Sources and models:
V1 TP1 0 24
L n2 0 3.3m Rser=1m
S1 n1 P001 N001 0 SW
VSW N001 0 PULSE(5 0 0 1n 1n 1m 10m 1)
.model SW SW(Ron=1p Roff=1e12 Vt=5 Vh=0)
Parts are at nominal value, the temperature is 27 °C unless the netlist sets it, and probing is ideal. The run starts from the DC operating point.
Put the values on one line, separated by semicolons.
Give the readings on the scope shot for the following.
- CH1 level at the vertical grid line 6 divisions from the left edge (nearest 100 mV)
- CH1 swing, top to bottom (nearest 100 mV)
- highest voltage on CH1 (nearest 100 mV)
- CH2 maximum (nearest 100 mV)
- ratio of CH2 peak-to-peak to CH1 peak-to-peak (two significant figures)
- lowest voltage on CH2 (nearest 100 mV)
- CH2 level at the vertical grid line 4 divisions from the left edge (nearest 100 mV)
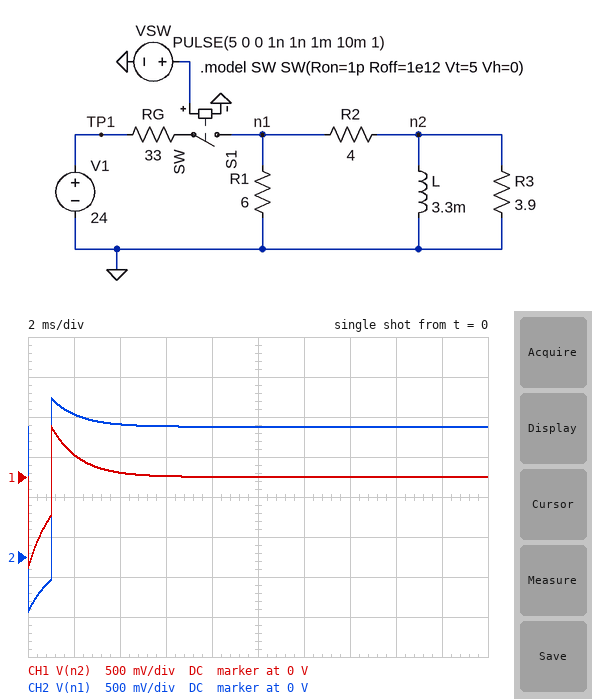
0 V; 1.8 V; 600 mV; 2.0 V; 1.5; -700 mV; 1.6 V
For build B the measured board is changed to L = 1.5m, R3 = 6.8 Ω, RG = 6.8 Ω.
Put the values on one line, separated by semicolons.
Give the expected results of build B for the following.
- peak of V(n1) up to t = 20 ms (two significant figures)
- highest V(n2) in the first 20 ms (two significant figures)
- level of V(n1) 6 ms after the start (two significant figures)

8.5 V; 5.1 V; 6.3 V
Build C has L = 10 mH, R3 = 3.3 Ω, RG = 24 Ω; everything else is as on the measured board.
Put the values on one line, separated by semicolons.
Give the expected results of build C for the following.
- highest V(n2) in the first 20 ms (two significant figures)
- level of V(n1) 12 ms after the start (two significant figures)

290 mV; 2.2 V
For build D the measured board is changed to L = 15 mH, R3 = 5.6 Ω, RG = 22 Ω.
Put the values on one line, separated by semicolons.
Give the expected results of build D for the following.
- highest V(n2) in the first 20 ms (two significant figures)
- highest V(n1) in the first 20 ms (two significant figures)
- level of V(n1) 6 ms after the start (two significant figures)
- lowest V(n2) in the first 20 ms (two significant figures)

430 mV; 2.6 V; 2.4 V; -2.1 V
